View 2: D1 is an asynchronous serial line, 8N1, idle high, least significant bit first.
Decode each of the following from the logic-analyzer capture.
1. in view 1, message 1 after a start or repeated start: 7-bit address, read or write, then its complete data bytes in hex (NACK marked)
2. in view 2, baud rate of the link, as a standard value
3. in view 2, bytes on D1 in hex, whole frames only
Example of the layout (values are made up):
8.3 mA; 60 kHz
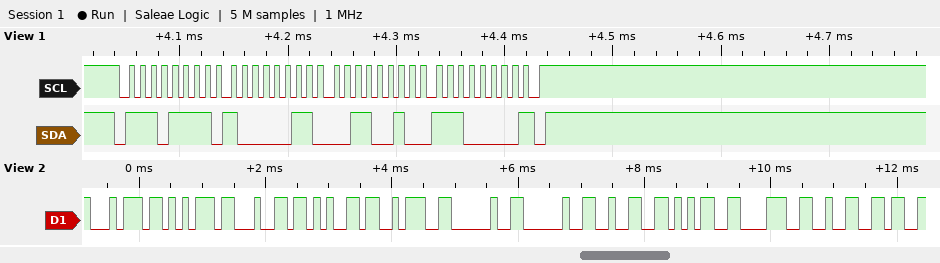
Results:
0x77 read: 83 32 E0 NACK; 9600 baud; 0x74 0x75 0x64 0x65 0x3A 0x20 0x20 0x32 0x35 0x38 0x32
